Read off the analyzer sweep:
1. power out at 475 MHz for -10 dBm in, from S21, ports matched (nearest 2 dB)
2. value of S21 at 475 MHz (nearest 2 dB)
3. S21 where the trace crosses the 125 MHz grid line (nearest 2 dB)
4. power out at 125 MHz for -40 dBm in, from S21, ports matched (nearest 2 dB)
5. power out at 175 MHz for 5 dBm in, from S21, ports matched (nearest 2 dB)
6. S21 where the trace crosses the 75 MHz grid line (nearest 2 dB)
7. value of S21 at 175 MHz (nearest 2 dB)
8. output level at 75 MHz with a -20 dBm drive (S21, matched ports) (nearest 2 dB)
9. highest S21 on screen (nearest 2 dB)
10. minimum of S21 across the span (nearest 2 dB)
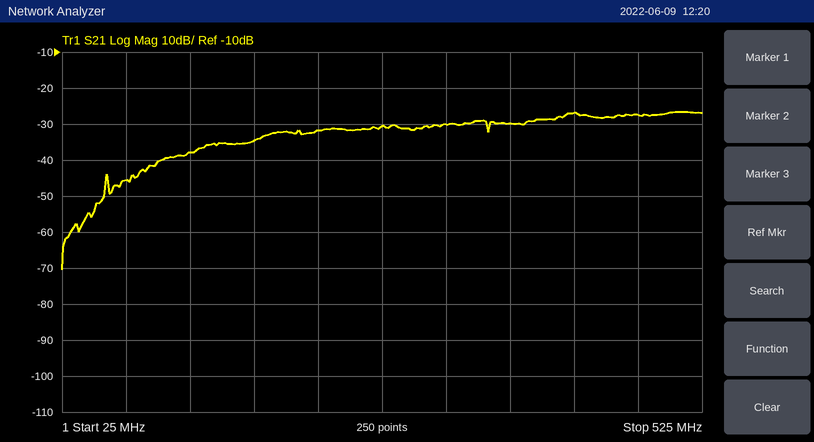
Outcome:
-38 dBm
-28 dB
-38 dB
-78 dBm
-30 dBm
-46 dB
-34 dB
-66 dBm
-26 dB
-70 dB
